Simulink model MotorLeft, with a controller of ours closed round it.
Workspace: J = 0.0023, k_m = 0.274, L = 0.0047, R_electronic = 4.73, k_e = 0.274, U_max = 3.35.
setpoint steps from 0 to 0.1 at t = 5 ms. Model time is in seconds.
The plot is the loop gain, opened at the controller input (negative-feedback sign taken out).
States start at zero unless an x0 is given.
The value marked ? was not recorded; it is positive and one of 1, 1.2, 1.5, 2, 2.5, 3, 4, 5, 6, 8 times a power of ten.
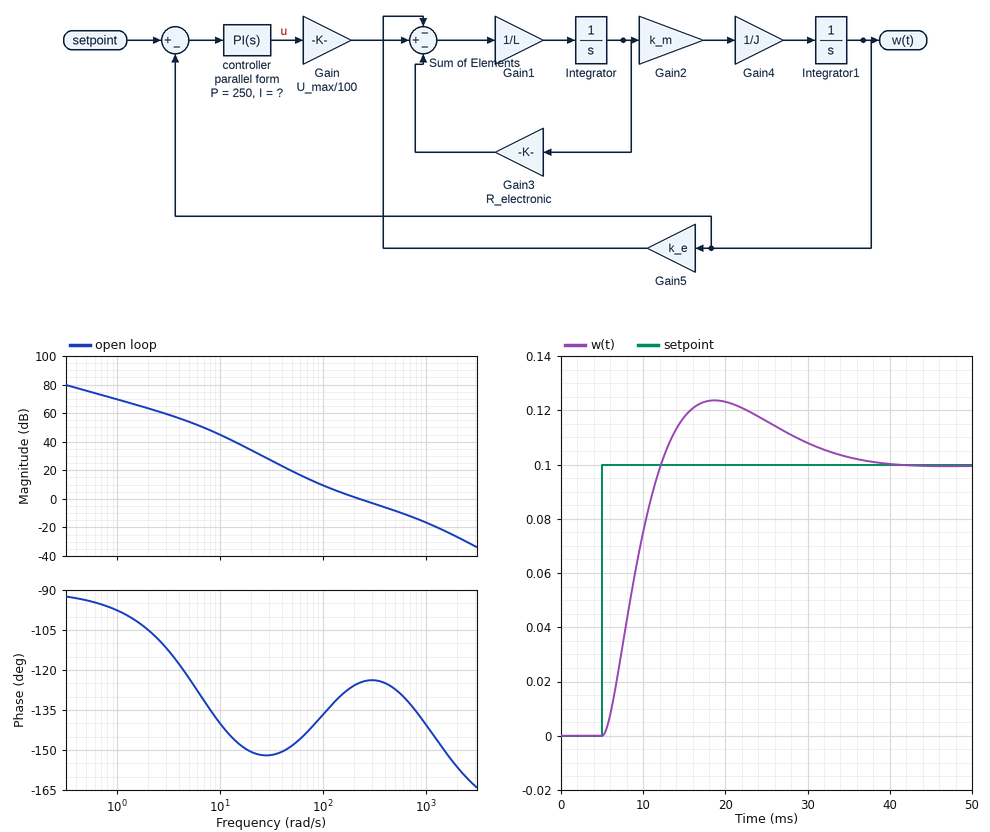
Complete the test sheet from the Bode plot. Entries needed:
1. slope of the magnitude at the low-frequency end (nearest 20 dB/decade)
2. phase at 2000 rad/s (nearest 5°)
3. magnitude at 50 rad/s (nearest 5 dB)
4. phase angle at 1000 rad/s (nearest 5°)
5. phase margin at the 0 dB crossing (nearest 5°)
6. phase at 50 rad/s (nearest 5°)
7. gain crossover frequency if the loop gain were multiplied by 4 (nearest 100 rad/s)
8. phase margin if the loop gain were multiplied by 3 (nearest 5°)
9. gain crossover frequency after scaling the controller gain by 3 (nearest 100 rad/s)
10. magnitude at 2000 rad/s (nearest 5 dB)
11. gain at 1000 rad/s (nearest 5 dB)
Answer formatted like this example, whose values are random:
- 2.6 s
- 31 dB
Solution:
- -20 dB/decade
- -155°
- 20 dB
- -140°
- 55°
- -150°
- 700 rad/s
- 50°
- 600 rad/s
- -25 dB
- -15 dB
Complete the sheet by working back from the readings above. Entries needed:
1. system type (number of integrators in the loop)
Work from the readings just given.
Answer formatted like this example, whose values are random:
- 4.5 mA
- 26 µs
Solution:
- 1
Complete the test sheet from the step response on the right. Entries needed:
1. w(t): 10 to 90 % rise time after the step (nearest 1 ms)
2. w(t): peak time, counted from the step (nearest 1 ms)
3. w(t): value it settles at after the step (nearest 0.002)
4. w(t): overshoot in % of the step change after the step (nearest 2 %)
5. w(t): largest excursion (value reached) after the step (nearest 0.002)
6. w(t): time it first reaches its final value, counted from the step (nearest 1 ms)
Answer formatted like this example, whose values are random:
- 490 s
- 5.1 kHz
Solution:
- 5 ms
- 14 ms
- 0.100
- 24 %
- 0.124
- 7 ms
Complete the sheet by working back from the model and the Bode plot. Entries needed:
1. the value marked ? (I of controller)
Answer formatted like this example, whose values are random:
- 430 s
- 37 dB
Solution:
- 25000
